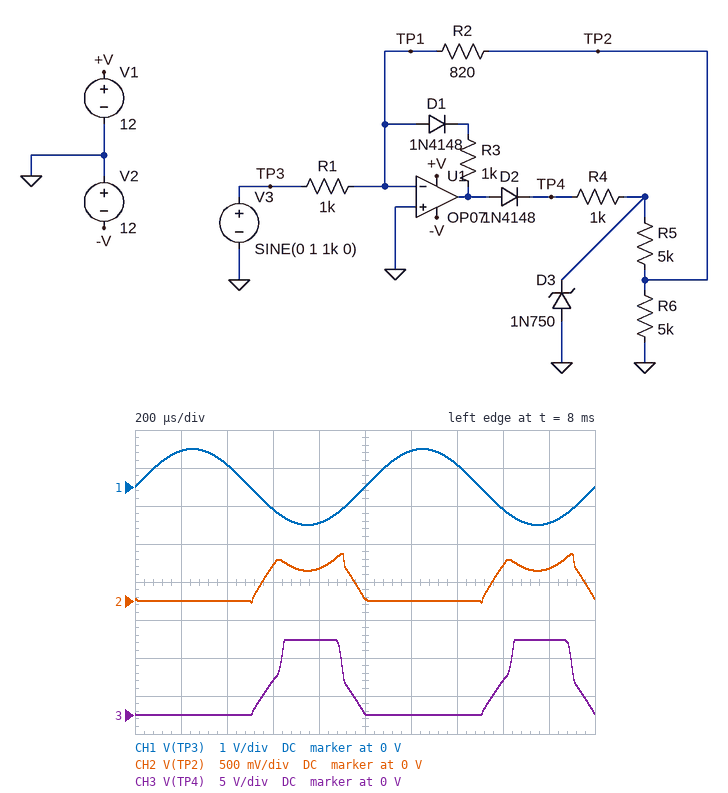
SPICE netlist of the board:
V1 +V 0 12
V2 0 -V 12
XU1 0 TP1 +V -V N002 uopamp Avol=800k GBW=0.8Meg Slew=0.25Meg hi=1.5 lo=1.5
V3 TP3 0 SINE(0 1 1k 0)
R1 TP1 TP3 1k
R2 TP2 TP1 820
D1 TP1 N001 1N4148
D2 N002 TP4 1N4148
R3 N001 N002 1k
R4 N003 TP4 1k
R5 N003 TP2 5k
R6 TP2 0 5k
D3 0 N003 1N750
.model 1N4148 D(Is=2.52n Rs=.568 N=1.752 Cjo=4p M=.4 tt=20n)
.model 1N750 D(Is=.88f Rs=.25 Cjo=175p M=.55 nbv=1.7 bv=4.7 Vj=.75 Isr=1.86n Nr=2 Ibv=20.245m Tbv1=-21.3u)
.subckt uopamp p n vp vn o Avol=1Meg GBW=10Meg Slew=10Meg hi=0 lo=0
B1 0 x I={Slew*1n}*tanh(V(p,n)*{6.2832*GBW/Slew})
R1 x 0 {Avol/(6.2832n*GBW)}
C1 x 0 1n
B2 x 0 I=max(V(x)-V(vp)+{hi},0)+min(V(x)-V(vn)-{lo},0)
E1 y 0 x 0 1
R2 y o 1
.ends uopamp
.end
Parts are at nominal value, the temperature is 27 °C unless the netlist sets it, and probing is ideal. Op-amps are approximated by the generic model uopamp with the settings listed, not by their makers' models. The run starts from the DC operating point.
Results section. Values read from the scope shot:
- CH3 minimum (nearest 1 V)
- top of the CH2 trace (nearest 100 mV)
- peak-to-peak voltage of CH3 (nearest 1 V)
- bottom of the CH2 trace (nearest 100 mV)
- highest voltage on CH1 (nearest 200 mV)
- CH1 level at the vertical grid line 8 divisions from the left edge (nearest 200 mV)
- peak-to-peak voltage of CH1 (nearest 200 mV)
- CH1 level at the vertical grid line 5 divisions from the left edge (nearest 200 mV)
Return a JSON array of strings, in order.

["0 V", "600 mV", "10 V", "0 V", "1.0 V", "-600 mV", "2.0 V", "0 V"]
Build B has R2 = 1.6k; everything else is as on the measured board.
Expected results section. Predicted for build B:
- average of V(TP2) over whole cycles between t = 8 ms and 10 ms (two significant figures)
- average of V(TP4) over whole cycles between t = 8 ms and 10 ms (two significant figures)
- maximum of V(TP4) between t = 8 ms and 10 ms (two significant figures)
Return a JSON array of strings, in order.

["330 mV", "3.6 V", "9.8 V"]
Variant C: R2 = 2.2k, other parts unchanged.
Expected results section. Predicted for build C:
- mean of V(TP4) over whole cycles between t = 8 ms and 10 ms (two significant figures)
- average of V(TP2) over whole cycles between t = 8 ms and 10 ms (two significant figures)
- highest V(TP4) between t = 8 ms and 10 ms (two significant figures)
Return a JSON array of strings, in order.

["3.8 V", "410 mV", "9.8 V"]
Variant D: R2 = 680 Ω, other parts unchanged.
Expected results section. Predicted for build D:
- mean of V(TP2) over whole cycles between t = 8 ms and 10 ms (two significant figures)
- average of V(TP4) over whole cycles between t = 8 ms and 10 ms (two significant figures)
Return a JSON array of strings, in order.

["160 mV", "3.1 V"]
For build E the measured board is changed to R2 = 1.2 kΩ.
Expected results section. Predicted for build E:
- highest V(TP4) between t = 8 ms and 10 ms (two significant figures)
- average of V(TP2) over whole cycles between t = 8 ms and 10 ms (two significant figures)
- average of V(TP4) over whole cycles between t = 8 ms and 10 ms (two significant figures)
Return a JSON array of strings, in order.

["9.8 V", "260 mV", "3.4 V"]
